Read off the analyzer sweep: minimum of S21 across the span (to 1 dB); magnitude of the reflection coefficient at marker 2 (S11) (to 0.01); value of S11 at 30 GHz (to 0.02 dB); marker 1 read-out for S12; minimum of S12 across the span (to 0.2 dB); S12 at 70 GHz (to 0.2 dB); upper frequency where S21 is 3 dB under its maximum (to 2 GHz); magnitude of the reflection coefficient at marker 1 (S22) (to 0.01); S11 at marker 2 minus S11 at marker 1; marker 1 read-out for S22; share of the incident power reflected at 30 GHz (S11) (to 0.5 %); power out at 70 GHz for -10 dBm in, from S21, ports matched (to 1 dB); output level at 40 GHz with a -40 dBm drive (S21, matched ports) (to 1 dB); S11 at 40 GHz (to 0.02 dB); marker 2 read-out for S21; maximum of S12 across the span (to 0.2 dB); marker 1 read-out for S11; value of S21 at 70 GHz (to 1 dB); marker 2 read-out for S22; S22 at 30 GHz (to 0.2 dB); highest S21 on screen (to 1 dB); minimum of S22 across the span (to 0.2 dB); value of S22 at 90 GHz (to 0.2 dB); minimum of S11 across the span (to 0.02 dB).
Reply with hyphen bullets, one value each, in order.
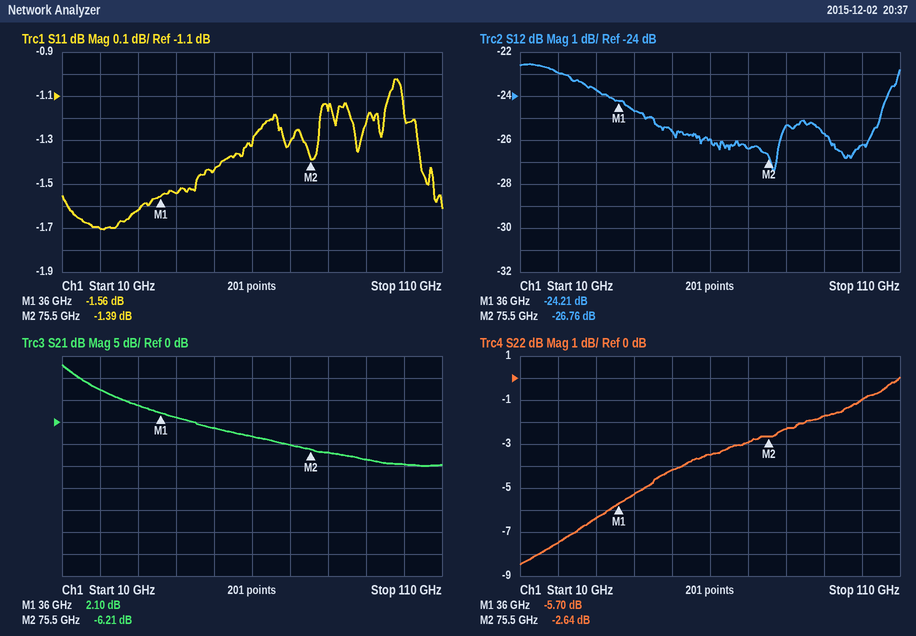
- -10 dB
- 0.85
- -1.62 dB
- -24.21 dB
- -27.4 dB
- -26.4 dB
- 14 GHz
- 0.52
- 0.17 dB
- -5.70 dB
- 69.0 %
- -15 dBm
- -39 dBm
- -1.54 dB
- -6.21 dB
- -22.6 dB
- -1.56 dB
- -5 dB
- -2.64 dB
- -6.4 dB
- 13 dB
- -8.4 dB
- -1.8 dB
- -1.70 dB
